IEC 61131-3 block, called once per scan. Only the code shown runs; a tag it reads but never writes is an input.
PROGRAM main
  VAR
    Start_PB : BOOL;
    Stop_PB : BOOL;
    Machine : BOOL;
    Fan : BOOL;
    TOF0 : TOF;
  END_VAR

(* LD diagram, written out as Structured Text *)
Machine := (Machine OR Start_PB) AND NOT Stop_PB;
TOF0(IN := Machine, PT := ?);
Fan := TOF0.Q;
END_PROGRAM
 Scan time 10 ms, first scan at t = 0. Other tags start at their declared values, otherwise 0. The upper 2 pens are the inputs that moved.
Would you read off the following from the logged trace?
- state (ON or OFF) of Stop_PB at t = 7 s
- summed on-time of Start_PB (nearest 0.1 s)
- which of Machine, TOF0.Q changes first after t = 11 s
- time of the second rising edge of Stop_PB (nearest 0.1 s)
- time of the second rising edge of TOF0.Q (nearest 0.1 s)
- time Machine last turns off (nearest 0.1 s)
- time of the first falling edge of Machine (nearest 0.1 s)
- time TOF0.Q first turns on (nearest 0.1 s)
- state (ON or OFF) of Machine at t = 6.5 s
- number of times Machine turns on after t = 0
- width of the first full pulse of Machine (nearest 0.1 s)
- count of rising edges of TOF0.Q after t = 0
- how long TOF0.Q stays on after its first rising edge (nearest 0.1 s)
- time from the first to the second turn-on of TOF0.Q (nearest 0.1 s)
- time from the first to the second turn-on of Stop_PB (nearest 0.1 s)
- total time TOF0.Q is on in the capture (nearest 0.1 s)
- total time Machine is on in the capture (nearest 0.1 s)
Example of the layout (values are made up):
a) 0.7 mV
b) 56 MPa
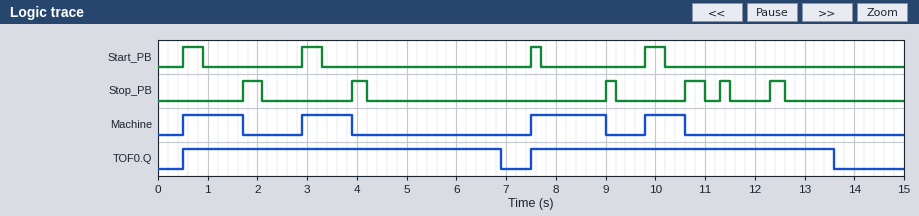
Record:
a) OFF
b) 1.4 s
c) TOF0.Q
d) 3.9 s
e) 7.5 s
f) 10.6 s
g) 1.7 s
h) 0.5 s
i) OFF
j) 4
k) 1.2 s
l) 2
m) 6.4 s
n) 7.0 s
o) 2.2 s
p) 12.5 s
q) 4.5 s
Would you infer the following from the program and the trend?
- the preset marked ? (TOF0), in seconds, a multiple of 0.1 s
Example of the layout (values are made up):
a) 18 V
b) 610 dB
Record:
a) 3.0 s
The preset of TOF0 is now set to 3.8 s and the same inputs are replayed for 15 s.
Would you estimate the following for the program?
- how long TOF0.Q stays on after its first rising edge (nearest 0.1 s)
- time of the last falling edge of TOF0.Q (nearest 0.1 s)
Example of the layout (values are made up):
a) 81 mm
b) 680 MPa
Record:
a) 13.9 s
b) 14.4 s
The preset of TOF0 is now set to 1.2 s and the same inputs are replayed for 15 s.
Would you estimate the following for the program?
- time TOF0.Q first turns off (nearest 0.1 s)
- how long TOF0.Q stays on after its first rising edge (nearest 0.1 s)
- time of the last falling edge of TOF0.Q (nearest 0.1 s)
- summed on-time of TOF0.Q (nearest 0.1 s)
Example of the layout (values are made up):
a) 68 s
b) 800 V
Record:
a) 5.1 s
b) 4.6 s
c) 11.8 s
d) 8.9 s
